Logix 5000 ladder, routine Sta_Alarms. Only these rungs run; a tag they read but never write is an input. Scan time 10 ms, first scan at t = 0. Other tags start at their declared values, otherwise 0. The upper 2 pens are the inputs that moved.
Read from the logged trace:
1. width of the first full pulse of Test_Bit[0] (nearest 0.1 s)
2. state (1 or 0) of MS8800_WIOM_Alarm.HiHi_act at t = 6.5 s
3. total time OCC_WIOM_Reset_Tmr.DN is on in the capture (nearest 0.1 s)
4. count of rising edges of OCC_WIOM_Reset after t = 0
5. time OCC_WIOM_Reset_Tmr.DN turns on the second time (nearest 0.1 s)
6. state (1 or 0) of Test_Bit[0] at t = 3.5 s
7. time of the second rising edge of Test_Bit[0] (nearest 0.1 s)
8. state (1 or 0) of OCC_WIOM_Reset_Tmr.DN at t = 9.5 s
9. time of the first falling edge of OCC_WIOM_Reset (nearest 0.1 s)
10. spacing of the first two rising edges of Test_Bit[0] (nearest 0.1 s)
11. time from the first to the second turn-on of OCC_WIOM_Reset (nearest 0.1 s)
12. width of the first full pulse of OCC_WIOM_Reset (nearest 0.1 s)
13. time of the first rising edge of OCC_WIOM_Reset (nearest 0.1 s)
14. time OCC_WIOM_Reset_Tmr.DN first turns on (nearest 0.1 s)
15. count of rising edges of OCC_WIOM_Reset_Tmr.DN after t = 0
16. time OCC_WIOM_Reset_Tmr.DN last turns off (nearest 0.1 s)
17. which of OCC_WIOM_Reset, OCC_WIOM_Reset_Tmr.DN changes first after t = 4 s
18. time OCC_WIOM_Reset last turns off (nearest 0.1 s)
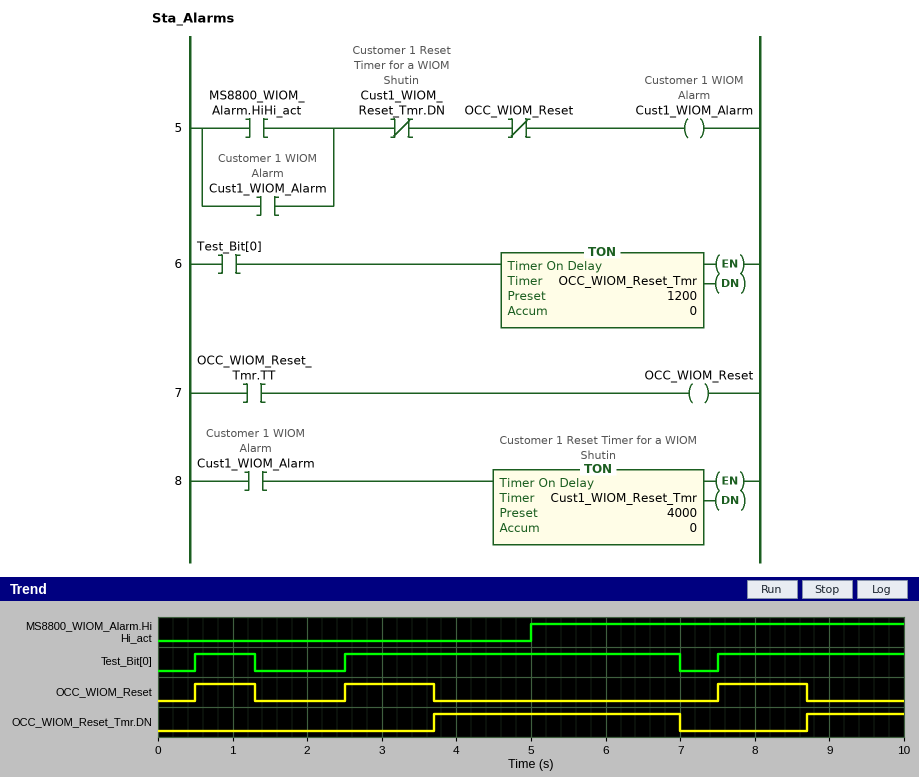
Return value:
0.8 s
1
4.6 s
3
8.7 s
1
2.5 s
1
1.3 s
2.0 s
2.0 s
0.8 s
0.5 s
3.7 s
2
7.0 s
OCC_WIOM_Reset_Tmr.DN
8.7 s
